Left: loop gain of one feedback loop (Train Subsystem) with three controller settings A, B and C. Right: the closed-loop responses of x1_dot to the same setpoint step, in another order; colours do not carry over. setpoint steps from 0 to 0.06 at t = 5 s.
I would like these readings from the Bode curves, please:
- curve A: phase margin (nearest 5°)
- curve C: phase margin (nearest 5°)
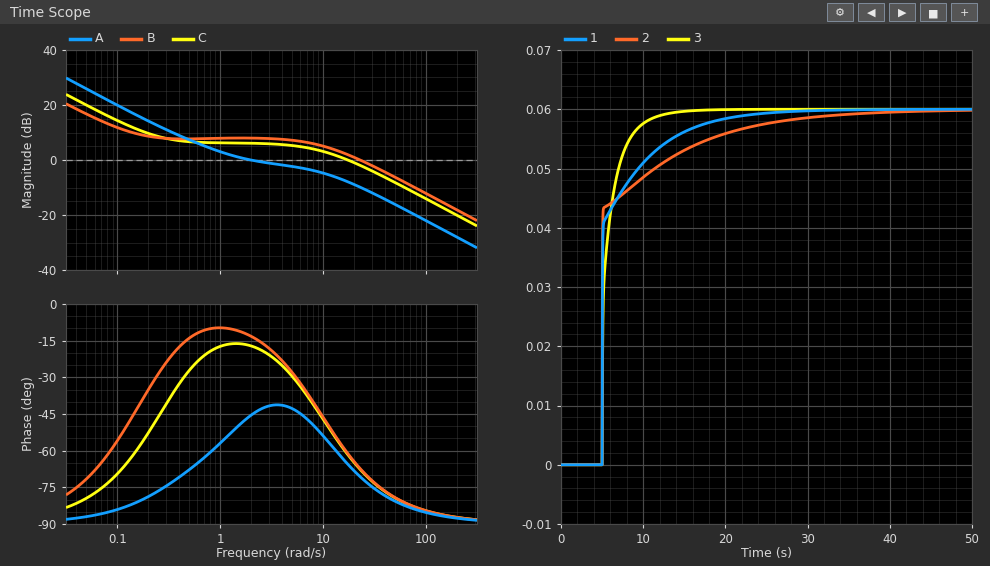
135°
120°
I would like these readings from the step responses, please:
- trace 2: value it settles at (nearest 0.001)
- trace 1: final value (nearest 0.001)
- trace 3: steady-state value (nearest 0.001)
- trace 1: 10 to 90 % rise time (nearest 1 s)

0.060
0.060
0.060
7 s
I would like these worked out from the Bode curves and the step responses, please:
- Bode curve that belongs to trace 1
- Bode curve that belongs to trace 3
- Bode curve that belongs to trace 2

C
A
B
